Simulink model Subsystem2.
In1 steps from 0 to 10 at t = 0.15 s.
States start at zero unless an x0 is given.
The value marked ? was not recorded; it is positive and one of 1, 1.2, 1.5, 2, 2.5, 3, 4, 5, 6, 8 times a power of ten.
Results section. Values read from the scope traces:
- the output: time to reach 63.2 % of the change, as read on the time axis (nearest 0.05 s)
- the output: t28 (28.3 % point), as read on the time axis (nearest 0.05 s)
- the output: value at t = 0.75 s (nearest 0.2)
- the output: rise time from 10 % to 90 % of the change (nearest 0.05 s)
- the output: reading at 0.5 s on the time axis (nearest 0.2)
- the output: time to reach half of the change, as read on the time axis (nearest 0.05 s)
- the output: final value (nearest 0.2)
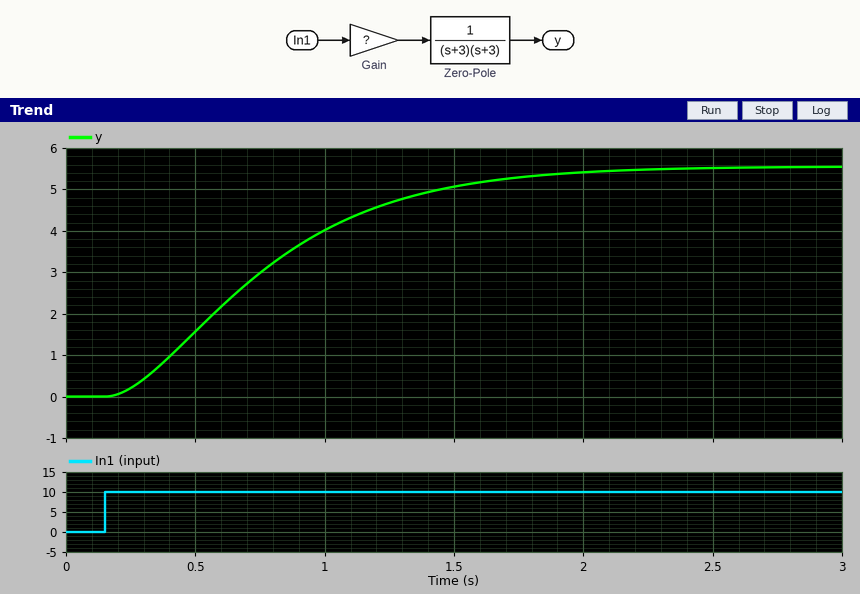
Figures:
0.85 s
0.50 s
3.0
1.10 s
1.6
0.70 s
5.6
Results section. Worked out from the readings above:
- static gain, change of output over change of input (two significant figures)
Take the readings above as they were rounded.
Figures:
0.56
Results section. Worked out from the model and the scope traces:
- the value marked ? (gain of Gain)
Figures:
5
